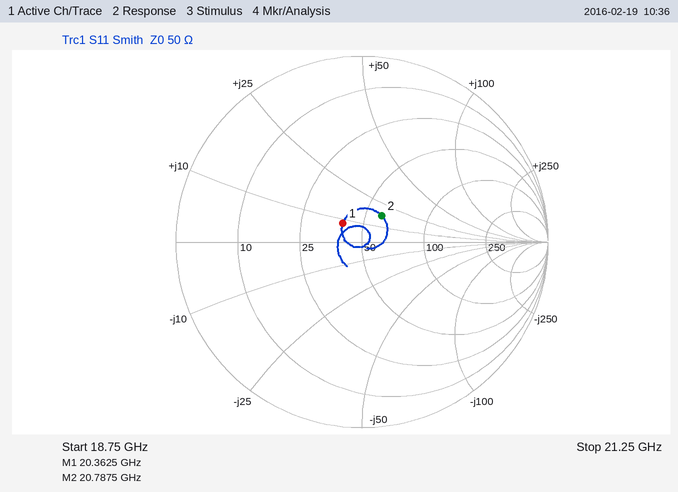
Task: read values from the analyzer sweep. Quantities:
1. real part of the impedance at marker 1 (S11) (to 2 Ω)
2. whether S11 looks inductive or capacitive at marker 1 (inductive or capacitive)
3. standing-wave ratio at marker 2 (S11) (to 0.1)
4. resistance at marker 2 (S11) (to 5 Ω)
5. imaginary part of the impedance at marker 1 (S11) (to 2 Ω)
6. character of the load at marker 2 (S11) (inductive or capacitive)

40 Ω
inductive
1.4
60 Ω
+8 Ω
inductive
